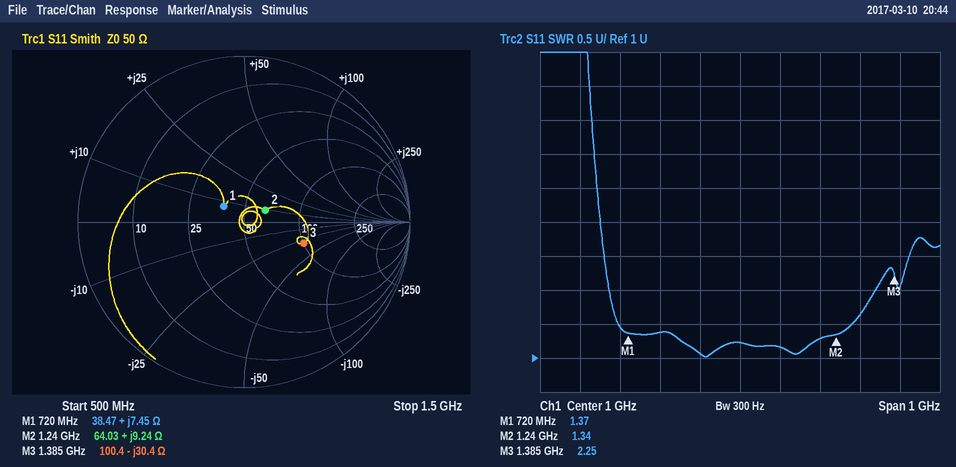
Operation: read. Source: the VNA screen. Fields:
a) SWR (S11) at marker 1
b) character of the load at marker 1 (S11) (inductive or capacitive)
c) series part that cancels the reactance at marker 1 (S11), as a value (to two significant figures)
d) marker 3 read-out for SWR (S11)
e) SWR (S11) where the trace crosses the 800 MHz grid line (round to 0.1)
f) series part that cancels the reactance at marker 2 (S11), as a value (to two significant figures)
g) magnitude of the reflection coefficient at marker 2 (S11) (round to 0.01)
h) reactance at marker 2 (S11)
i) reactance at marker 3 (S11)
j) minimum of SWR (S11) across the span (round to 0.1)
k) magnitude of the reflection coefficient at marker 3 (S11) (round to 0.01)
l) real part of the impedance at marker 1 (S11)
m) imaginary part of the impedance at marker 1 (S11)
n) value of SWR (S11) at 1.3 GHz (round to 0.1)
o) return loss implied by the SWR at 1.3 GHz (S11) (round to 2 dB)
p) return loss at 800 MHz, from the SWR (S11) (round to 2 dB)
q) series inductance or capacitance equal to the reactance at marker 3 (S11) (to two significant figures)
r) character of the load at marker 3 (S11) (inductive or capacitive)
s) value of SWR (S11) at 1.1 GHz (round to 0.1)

1.37
inductive
30 pF
2.25
1.4
14 pF
0.15
+9.24 Ω
-30.4 Ω
1.0
0.38
38.47 Ω
+7.45 Ω
1.6
12 dB
16 dB
3.8 pF
capacitive
1.2
